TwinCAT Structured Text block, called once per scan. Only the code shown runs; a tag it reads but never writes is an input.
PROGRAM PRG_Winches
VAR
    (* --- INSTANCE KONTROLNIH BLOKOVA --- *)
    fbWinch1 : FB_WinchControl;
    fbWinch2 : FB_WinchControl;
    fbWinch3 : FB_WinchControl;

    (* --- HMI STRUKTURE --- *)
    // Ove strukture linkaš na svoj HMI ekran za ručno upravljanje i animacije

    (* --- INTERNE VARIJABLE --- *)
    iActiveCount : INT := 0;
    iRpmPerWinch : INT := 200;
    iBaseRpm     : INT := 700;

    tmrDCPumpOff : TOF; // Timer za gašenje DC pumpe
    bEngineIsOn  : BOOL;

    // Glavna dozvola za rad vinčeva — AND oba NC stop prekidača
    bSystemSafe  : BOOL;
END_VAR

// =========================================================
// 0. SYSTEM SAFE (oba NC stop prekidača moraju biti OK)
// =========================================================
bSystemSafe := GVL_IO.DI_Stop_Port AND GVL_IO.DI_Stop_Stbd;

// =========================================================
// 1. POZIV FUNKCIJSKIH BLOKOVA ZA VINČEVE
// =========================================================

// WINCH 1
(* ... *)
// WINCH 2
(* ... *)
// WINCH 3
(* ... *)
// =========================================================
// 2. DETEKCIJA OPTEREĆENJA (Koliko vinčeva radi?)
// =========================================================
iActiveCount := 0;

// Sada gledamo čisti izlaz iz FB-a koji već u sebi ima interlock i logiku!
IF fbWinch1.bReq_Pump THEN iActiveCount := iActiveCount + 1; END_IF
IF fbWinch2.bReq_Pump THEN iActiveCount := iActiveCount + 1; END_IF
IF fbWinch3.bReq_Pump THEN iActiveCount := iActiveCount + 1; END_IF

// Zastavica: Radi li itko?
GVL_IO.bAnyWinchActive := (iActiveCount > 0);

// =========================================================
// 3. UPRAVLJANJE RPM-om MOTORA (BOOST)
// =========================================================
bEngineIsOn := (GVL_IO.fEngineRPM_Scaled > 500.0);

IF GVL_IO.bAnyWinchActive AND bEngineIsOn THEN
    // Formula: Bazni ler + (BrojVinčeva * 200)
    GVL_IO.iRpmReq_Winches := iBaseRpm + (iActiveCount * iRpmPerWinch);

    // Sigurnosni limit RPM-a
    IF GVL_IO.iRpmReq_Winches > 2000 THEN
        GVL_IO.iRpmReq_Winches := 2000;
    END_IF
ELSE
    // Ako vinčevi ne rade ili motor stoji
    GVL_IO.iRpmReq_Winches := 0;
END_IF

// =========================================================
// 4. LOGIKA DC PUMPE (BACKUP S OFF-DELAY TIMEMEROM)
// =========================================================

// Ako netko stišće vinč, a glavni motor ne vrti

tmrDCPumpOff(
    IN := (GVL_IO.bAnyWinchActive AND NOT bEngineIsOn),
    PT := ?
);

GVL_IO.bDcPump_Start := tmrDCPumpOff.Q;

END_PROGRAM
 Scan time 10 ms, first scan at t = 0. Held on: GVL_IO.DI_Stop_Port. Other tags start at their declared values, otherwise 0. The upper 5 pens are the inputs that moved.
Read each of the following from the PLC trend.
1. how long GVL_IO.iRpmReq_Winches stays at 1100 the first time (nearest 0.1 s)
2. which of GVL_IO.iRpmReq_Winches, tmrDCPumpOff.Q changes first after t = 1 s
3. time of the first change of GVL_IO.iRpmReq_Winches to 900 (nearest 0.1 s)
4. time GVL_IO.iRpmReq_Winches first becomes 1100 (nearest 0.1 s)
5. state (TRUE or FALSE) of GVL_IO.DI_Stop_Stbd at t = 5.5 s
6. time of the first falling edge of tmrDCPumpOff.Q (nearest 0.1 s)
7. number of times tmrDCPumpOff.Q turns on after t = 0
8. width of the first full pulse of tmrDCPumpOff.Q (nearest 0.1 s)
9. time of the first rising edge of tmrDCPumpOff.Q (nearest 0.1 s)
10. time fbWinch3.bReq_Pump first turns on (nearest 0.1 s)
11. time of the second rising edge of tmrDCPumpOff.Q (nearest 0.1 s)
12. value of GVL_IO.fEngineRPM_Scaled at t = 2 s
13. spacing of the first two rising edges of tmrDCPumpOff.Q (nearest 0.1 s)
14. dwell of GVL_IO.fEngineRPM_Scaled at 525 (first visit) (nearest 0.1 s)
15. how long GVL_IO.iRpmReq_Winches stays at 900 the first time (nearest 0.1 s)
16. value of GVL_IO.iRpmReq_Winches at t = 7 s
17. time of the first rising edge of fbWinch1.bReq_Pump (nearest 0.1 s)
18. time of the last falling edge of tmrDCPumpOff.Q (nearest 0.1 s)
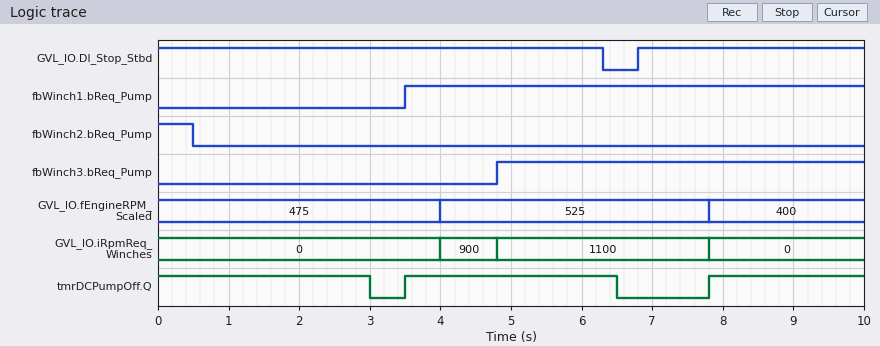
3.0 s
tmrDCPumpOff.Q
4.0 s
4.8 s
TRUE
3.0 s
2
3.0 s
3.5 s
4.8 s
7.8 s
475
4.3 s
3.8 s
0.8 s
1100
3.5 s
6.5 s
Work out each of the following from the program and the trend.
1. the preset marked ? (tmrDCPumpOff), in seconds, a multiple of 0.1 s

2.5 s
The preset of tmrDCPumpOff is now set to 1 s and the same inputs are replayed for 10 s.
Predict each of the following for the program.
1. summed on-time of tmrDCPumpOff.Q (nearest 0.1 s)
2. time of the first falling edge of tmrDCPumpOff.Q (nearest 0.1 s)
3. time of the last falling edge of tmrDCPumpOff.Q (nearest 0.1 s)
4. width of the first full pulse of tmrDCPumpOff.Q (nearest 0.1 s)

5.2 s
1.5 s
5.0 s
1.5 s
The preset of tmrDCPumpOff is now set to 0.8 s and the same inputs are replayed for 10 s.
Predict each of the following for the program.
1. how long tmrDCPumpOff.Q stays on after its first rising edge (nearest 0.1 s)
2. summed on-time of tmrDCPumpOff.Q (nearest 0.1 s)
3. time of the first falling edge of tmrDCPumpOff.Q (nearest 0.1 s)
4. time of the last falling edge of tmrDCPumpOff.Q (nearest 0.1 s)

1.3 s
4.8 s
1.3 s
4.8 s
